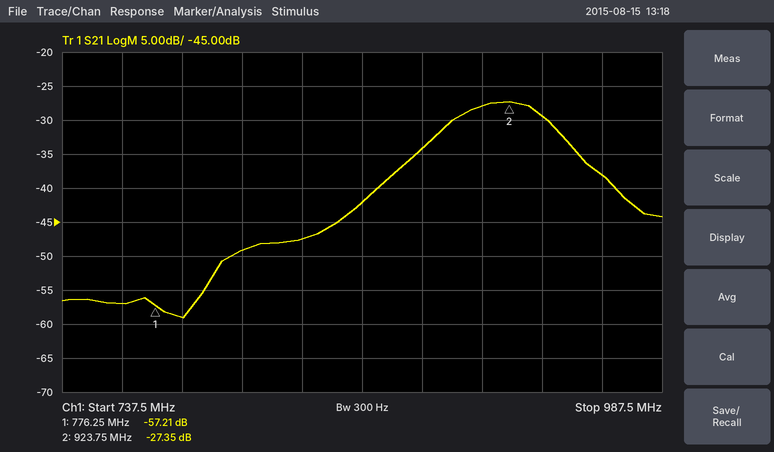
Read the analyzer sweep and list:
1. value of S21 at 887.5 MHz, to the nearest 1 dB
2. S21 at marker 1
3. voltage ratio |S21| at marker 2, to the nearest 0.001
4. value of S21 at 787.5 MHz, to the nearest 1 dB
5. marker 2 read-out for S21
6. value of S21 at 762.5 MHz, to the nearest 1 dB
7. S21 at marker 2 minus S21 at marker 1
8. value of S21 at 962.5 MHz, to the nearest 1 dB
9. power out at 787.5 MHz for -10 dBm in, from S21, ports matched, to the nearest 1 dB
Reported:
-34 dB
-57.21 dB
0.043
-59 dB
-27.35 dB
-57 dB
29.86 dB
-38 dB
-69 dBm
